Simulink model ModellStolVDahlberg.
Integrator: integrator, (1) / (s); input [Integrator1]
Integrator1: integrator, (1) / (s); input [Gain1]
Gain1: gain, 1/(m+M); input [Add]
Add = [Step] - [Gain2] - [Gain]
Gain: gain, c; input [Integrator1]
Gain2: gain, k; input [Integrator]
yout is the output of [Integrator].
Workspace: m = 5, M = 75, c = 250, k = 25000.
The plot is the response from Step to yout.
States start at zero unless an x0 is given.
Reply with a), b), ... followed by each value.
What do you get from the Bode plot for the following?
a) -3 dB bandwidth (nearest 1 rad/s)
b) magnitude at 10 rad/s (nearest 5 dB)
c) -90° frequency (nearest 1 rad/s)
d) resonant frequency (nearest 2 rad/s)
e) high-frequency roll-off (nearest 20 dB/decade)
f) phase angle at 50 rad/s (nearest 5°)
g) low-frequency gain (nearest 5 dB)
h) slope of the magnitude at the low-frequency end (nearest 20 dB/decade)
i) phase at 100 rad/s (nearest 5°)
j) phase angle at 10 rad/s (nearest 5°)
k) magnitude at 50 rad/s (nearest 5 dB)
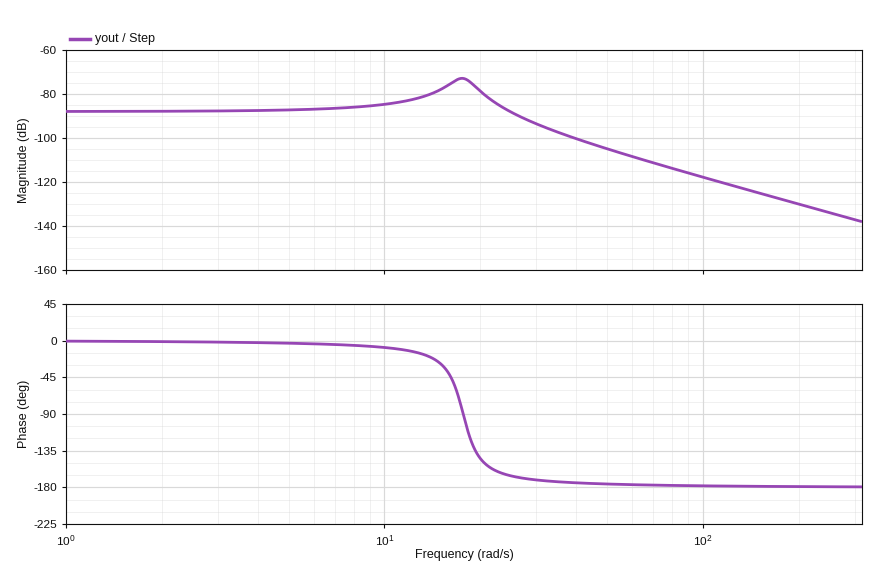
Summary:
a) 27 rad/s
b) -85 dB
c) 18 rad/s
d) 18 rad/s
e) -40 dB/decade
f) -175°
g) -90 dB
h) 0 dB/decade
i) -180°
j) -10°
k) -105 dB
